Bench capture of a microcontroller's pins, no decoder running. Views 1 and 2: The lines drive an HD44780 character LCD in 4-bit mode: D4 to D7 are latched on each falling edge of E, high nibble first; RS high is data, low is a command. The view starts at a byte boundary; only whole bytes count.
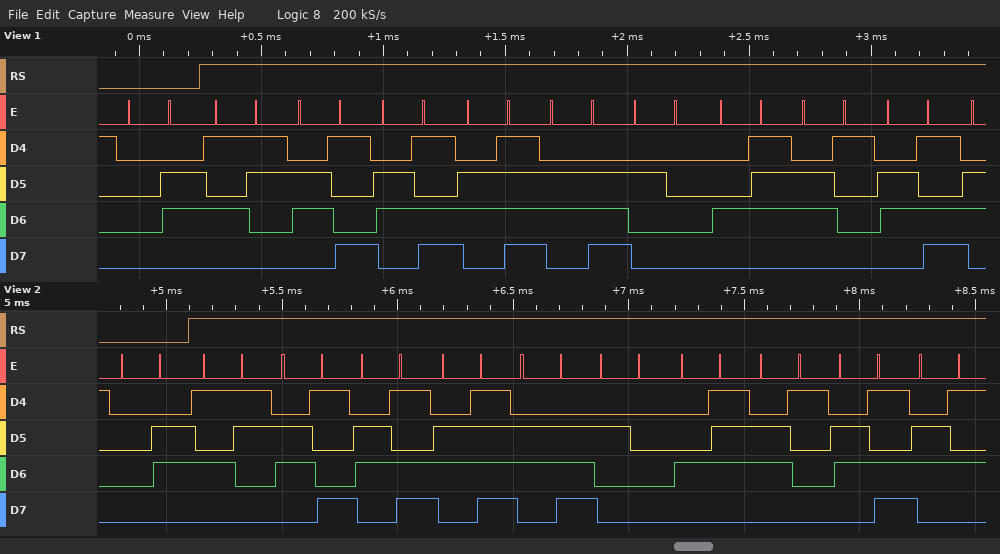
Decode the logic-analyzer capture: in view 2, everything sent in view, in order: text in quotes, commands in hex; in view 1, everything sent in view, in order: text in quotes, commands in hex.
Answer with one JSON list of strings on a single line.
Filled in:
["0x06 \"Simon Game\"", "0x06 \"Simon Gam\""]
